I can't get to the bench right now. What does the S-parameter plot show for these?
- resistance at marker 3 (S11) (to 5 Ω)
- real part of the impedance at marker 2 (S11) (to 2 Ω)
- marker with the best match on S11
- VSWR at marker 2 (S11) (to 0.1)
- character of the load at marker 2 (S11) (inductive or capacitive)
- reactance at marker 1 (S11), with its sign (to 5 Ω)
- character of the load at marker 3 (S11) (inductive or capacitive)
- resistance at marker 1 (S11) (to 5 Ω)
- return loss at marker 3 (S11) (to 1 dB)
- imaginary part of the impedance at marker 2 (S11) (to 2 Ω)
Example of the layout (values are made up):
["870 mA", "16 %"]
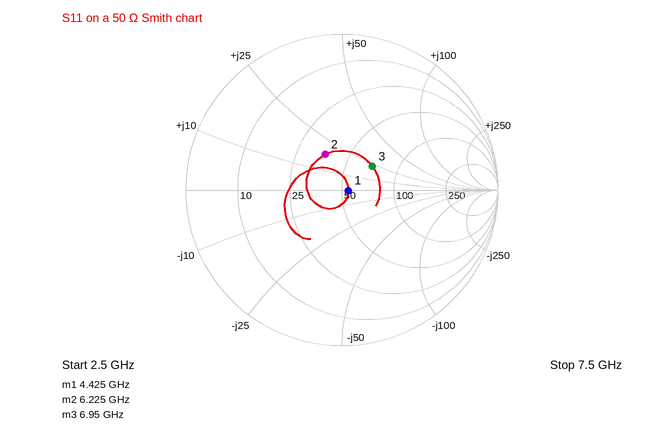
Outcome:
["70 Ω", "36 Ω", "marker 1", "1.7", "inductive", "0 Ω", "inductive", "55 Ω", "12 dB", "+18 Ω"]
